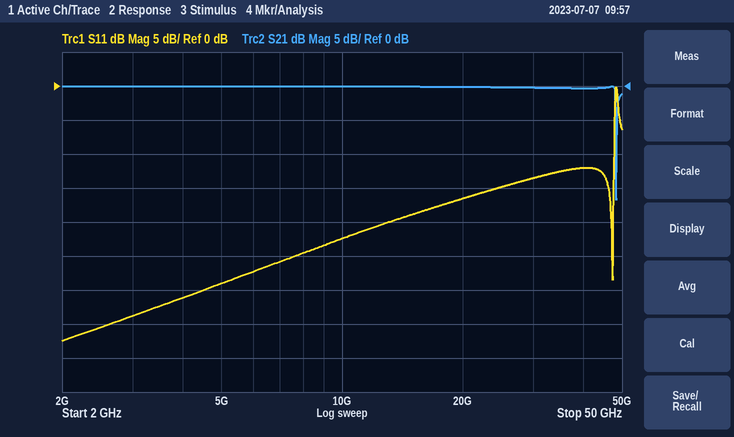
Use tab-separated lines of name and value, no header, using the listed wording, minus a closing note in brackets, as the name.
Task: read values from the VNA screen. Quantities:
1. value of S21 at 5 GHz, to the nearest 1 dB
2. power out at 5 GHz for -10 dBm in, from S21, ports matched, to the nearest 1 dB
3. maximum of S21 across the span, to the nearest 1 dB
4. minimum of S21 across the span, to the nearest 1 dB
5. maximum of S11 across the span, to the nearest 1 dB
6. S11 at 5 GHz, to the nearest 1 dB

value of S21 at 5 GHz, to the nearest 1 dB	0 dB
power out at 5 GHz for -10 dBm in, from S21, ports matched, to the nearest 1 dB	-10 dBm
maximum of S21 across the span, to the nearest 1 dB	0 dB
minimum of S21 across the span, to the nearest 1 dB	-17 dB
maximum of S11 across the span, to the nearest 1 dB	0 dB
S11 at 5 GHz, to the nearest 1 dB	-29 dB
